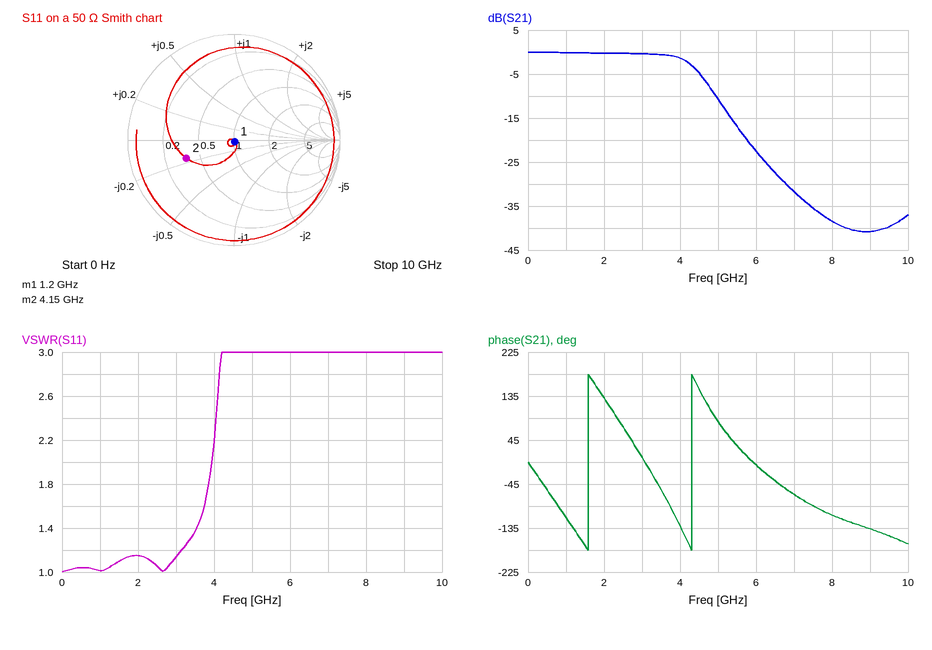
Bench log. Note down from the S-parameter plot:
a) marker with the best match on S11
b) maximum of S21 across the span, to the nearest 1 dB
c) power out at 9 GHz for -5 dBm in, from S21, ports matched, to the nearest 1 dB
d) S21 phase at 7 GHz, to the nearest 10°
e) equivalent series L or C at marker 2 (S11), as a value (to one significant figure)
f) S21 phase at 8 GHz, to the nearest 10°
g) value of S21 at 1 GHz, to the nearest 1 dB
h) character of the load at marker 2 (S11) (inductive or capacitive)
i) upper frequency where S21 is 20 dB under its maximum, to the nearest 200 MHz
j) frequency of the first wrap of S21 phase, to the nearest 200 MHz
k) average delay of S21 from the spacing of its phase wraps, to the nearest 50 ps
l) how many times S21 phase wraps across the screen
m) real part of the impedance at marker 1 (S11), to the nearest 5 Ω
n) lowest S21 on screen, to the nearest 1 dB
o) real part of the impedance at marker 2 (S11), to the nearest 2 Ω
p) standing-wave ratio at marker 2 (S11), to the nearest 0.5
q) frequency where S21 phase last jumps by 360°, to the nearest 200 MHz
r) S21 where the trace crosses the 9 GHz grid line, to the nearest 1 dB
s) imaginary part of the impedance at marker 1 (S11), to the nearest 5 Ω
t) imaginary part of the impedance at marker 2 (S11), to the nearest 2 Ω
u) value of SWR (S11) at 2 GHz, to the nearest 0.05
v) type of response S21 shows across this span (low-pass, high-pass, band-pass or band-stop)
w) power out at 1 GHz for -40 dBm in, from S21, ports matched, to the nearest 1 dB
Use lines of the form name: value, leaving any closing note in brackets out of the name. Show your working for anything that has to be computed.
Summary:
marker with the best match on S11: marker 1
maximum of S21 across the span, to the nearest 1 dB: 0 dB
power out at 9 GHz for -5 dBm in, from S21, ports matched, to the nearest 1 dB: -5 dBm + (-41 dB) = -46 dBm
S21 phase at 7 GHz, to the nearest 10°: -70°
equivalent series L or C at marker 2 (S11), as a value: C = 1/(2π × 4.15 GHz × 8 Ω) ≈ 5 pF
S21 phase at 8 GHz, to the nearest 10°: -110°
value of S21 at 1 GHz, to the nearest 1 dB: 0 dB
character of the load at marker 2 (S11): capacitive
upper frequency where S21 is 20 dB under its maximum, to the nearest 200 MHz: 5.8 GHz
frequency of the first wrap of S21 phase, to the nearest 200 MHz: 1.6 GHz
average delay of S21 from the spacing of its phase wraps, to the nearest 50 ps: 1 cycle / (4.4 GHz − 1.6 GHz) ≈ 357 ps, so 350 ps to the nearest 50 ps
how many times S21 phase wraps across the screen: 2
real part of the impedance at marker 1 (S11), to the nearest 5 Ω: 50 Ω
lowest S21 on screen, to the nearest 1 dB: -41 dB
real part of the impedance at marker 2 (S11), to the nearest 2 Ω: 18 Ω
standing-wave ratio at marker 2 (S11), to the nearest 0.5: 3.0
frequency where S21 phase last jumps by 360°, to the nearest 200 MHz: 4.4 GHz
S21 where the trace crosses the 9 GHz grid line, to the nearest 1 dB: -41 dB
imaginary part of the impedance at marker 1 (S11), to the nearest 5 Ω: 0 Ω
imaginary part of the impedance at marker 2 (S11), to the nearest 2 Ω: -8 Ω
value of SWR (S11) at 2 GHz, to the nearest 0.05: 1.15
type of response S21 shows across this span: low-pass
power out at 1 GHz for -40 dBm in, from S21, ports matched, to the nearest 1 dB: -40 dBm + (0 dB) = -40 dBm
